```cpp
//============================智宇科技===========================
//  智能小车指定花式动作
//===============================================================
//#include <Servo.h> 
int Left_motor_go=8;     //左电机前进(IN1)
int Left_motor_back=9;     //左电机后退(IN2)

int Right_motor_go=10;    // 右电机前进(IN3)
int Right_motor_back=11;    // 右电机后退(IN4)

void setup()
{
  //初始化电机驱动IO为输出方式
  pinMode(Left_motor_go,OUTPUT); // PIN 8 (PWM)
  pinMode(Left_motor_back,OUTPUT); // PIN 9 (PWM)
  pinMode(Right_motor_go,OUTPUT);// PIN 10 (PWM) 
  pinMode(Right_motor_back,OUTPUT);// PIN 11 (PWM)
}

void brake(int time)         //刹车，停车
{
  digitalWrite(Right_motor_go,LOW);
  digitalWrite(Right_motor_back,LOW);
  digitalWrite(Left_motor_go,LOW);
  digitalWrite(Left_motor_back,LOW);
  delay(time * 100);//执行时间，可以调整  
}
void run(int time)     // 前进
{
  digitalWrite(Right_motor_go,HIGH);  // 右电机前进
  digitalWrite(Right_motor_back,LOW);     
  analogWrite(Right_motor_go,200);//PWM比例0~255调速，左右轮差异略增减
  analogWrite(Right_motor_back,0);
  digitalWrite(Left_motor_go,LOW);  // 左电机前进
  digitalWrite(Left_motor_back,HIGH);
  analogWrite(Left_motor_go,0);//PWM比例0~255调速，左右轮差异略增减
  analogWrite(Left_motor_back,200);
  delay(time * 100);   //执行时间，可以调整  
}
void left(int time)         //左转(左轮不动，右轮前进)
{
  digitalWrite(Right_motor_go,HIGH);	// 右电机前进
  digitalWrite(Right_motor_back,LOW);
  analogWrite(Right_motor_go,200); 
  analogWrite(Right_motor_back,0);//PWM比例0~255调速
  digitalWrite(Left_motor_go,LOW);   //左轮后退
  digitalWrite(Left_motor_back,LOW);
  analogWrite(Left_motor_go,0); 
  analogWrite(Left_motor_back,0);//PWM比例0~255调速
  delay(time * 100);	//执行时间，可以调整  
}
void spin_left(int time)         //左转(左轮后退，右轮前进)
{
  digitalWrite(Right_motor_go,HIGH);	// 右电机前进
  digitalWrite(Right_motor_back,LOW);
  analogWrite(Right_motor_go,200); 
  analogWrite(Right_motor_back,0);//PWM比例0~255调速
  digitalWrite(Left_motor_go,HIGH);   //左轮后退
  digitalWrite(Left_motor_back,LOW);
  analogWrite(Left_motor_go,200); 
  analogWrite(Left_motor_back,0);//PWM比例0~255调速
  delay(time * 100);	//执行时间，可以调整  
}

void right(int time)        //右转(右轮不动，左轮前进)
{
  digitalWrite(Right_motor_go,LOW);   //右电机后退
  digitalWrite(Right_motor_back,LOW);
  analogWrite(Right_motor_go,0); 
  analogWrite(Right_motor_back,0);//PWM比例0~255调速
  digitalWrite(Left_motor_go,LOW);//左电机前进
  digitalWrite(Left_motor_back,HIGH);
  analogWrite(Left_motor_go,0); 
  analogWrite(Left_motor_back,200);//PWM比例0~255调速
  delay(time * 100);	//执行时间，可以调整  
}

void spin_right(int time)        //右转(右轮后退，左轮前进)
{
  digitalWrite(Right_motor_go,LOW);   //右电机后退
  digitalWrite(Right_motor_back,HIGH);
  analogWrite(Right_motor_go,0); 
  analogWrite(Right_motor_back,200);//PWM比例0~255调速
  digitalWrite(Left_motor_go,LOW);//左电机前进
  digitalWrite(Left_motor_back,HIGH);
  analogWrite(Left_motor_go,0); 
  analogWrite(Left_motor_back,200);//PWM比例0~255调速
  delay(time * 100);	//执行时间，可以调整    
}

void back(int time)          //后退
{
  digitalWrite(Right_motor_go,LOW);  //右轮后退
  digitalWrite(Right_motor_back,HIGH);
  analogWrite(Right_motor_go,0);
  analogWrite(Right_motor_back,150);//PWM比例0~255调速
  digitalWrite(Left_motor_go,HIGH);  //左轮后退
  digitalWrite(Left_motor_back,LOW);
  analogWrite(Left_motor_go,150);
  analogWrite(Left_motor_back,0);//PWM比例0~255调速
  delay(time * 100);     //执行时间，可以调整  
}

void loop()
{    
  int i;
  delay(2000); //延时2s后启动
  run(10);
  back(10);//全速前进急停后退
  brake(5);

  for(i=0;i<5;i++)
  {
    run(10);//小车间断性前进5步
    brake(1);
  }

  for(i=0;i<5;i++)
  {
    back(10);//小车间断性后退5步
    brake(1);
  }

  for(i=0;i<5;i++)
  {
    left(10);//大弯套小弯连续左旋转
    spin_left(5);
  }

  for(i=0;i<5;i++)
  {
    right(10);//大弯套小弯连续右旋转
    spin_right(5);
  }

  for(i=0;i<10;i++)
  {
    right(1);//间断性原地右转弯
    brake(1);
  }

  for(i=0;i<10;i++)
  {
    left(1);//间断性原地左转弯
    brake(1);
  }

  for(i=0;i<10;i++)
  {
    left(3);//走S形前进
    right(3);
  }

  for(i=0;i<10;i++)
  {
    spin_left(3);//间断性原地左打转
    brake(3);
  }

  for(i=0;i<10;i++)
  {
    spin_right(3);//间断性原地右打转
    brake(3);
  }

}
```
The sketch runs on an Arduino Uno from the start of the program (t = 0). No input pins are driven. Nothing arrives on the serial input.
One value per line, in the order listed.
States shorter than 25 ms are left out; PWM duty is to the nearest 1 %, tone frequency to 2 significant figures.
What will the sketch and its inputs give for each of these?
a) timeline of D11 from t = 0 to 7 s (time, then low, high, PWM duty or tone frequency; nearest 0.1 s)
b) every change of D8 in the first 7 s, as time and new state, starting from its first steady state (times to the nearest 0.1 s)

0 s low; 3 s PWM 59 %; 4 s low
0 s low; 3 s high; 4 s low
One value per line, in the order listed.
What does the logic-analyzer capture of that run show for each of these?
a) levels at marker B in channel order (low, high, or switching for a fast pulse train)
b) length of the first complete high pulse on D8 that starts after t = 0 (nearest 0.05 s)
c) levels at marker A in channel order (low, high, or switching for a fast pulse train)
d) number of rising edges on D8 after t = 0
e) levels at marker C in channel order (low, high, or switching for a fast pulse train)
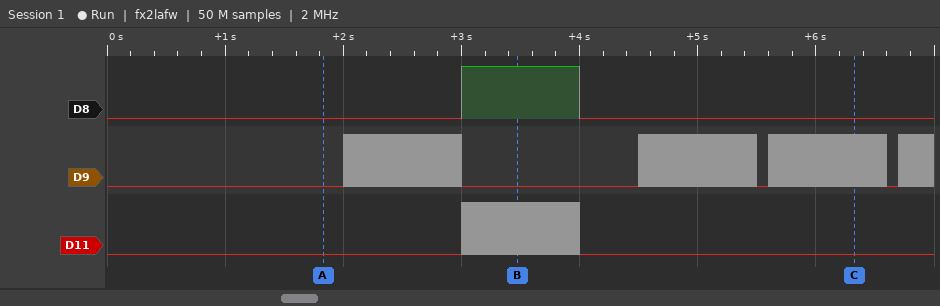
D8 high, D9 low, D11 switching
1.00 s
D8 low, D9 low, D11 low
1
D8 low, D9 switching, D11 low
